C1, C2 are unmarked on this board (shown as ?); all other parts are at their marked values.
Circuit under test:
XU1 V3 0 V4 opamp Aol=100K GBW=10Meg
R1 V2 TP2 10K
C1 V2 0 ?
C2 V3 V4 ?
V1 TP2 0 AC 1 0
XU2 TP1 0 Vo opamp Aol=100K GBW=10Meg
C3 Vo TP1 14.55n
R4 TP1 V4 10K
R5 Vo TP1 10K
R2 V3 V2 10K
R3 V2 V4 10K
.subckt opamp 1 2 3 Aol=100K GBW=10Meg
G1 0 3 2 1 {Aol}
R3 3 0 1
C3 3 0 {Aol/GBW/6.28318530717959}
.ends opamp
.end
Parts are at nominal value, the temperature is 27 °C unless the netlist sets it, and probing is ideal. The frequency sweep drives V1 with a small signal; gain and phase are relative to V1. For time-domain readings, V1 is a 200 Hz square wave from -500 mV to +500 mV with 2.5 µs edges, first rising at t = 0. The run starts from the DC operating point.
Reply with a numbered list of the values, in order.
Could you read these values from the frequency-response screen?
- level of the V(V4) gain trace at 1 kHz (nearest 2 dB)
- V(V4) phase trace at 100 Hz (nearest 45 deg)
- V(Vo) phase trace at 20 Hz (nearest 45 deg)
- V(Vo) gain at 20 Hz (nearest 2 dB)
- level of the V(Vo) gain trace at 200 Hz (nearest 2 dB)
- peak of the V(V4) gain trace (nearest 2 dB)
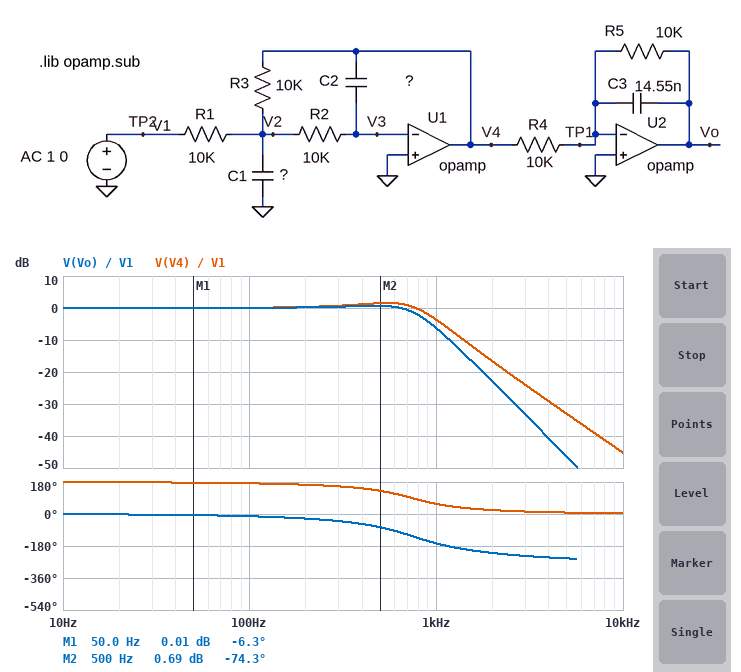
1. -4 dB
2. 180 deg
3. 0 deg
4. 0 dB
5. 0 dB
6. 2 dB
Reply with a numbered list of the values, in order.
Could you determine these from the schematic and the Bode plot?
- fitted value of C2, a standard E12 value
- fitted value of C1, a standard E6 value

1. 6.8 nF
2. 68 nF
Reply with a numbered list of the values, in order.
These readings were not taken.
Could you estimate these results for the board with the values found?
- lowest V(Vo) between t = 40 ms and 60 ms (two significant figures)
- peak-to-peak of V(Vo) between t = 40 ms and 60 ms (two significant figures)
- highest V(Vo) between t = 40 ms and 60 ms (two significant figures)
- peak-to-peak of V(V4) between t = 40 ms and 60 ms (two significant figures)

1. -640 mV
2. 1.3 V
3. 640 mV
4. 1.4 V
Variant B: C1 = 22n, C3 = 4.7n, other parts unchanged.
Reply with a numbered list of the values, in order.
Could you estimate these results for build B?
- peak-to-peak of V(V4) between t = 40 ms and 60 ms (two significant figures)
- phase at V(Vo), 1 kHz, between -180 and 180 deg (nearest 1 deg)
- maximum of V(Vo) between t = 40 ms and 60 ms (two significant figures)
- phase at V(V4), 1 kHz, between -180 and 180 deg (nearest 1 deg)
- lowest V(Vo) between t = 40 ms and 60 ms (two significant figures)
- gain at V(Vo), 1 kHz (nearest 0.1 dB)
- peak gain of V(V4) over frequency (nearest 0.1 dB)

1. 1.0 V
2. -89 deg
3. 510 mV
4. 108 deg
5. -510 mV
6. -2.9 dB
7. 0 dB
